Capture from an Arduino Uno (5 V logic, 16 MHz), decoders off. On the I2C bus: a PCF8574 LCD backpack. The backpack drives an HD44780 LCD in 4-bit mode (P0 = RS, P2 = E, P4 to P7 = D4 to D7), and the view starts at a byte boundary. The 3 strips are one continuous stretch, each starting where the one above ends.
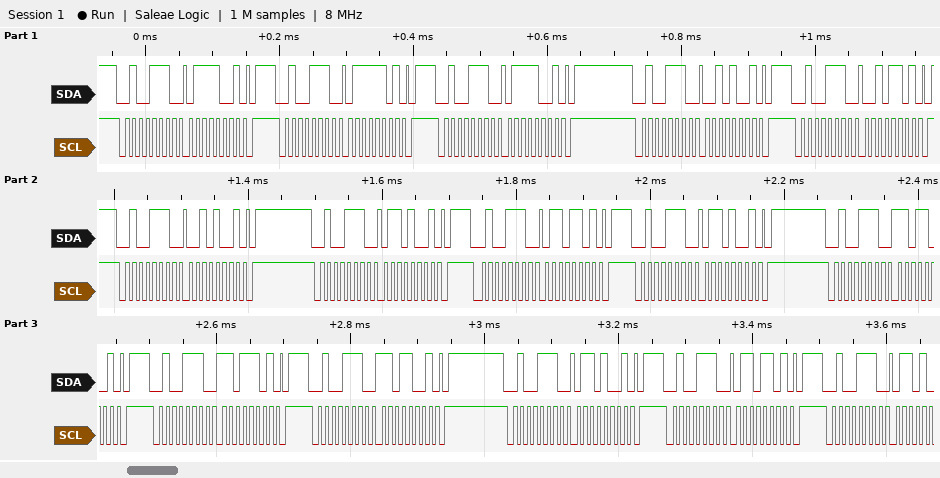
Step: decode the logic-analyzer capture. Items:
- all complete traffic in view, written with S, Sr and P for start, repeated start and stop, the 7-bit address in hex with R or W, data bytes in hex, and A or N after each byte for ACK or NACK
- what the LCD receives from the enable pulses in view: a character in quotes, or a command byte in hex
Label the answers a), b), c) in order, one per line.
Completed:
a) S 27W A 79 A P S 27W A 7D A P S 27W A 79 A P S 27W A 29 A P S 27W A 2D A P S 27W A 29 A P S 27W A 69 A P S 27W A 6D A P S 27W A 69 A P S 27W A D9 A P S 27W A DD A P S 27W A D9 A P S 27W A 69 A P S 27W A 6D A P S 27W A
b) 'r' 'm'
